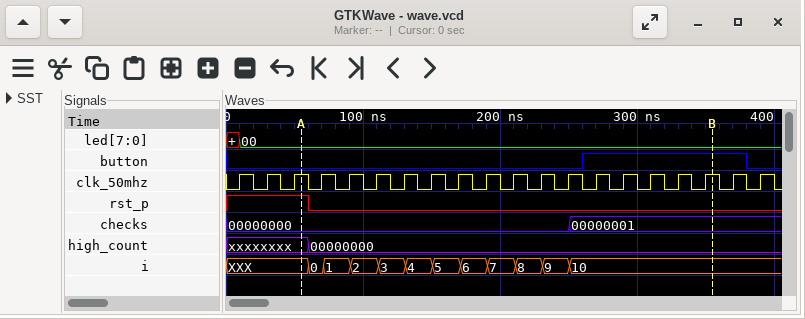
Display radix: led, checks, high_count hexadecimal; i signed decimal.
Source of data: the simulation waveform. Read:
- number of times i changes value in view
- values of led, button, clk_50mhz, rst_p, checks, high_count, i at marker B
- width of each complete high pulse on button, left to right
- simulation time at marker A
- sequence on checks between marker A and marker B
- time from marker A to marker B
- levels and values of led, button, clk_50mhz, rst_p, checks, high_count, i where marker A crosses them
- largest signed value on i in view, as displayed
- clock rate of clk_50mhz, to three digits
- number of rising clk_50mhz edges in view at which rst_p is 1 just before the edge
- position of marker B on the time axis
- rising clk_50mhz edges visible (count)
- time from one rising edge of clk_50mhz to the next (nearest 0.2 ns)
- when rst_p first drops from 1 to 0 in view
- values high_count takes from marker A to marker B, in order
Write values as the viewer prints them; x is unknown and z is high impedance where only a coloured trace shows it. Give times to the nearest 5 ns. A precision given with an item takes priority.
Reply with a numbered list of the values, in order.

1. 11
2. led=00, button=1, clk_50mhz=1, rst_p=0, checks=00000001, high_count=00000000, i=10
3. 120 ns
4. 55 ns
5. 00000000, 00000001
6. 300 ns
7. led=00, button=0, clk_50mhz=1, rst_p=1, checks=00000000, high_count=xxxxxxxx, i=XXX
8. 10
9. 50.0 MHz
10. 3
11. 355 ns
12. 20
13. 20 ns
14. 60 ns
15. xxxxxxxx, 00000000
